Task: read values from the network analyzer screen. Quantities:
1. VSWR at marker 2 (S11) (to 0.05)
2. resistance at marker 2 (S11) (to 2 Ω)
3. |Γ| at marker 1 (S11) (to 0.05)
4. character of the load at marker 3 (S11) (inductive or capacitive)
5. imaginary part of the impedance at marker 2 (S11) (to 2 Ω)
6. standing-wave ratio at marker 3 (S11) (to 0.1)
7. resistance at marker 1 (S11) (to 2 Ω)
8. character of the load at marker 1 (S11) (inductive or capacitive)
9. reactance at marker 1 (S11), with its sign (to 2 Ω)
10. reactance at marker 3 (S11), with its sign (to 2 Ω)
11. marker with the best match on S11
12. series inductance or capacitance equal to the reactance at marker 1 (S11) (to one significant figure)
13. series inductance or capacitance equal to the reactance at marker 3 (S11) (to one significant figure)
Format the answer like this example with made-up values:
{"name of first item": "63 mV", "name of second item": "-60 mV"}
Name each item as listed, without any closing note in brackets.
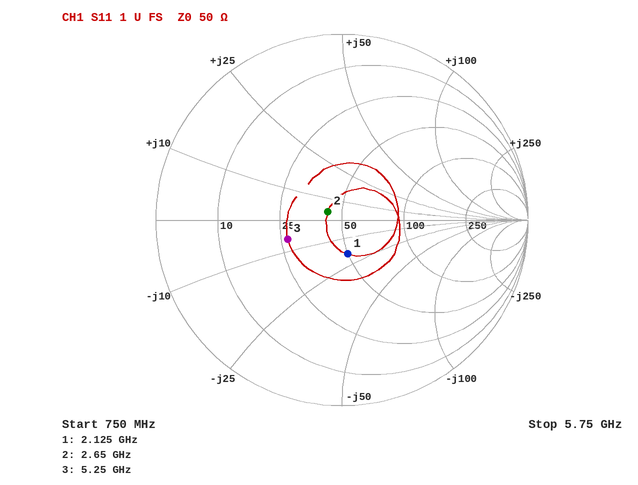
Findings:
{"VSWR at marker 2 (S11)": "1.20", "resistance at marker 2 (S11)": "42 Ω", "|Γ| at marker 1 (S11)": "0.20", "character of the load at marker 3 (S11)": "capacitive", "imaginary part of the impedance at marker 2 (S11)": "+4 Ω", "standing-wave ratio at marker 3 (S11)": "1.9", "resistance at marker 1 (S11)": "50 Ω", "character of the load at marker 1 (S11)": "capacitive", "reactance at marker 1 (S11), with its sign": "-18 Ω", "reactance at marker 3 (S11), with its sign": "-6 Ω", "marker with the best match on S11": "marker 2", "series inductance or capacitance equal to the reactance at marker 1 (S11)": "4 pF", "series inductance or capacitance equal to the reactance at marker 3 (S11)": "5 pF"}
